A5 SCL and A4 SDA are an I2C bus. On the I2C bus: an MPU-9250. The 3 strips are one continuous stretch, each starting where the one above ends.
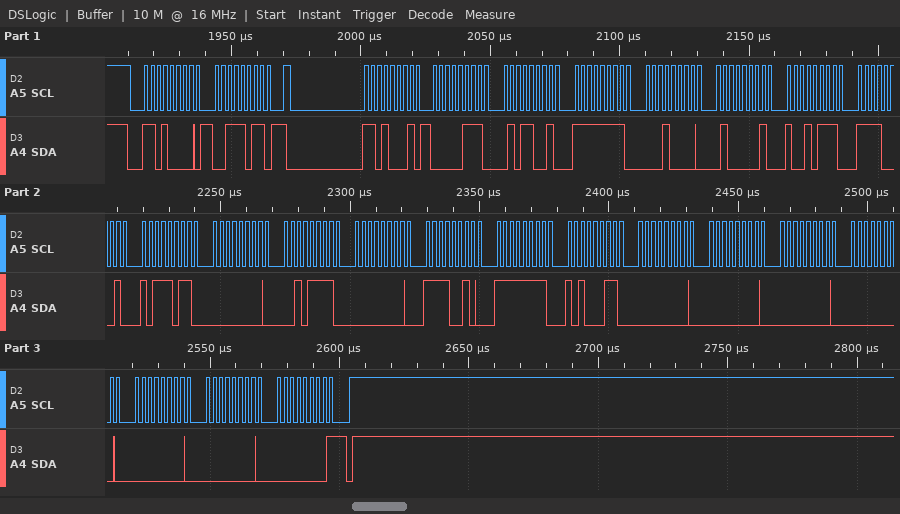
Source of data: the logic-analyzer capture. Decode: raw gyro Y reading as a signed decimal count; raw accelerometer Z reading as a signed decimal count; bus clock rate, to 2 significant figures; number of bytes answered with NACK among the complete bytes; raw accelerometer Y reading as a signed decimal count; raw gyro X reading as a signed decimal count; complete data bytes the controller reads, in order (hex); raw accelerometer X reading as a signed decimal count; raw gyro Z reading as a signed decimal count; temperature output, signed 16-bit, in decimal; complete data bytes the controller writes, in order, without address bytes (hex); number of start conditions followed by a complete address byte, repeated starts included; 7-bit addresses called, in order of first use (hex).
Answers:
242
16791
400 kHz
1
-240
47
07 59 FF 10 41 97 F1 BB 00 2F 00 F2 FF A3 00 00 00 00 00 00 00
1881
-93
-3653
3B
2
0x68
